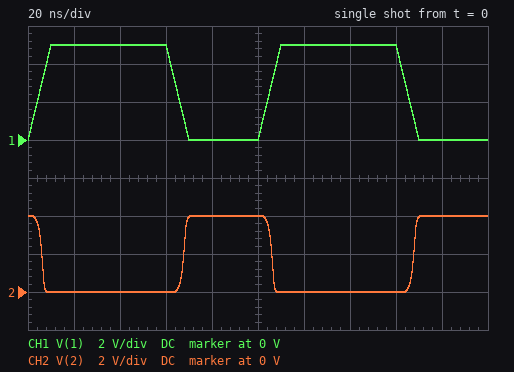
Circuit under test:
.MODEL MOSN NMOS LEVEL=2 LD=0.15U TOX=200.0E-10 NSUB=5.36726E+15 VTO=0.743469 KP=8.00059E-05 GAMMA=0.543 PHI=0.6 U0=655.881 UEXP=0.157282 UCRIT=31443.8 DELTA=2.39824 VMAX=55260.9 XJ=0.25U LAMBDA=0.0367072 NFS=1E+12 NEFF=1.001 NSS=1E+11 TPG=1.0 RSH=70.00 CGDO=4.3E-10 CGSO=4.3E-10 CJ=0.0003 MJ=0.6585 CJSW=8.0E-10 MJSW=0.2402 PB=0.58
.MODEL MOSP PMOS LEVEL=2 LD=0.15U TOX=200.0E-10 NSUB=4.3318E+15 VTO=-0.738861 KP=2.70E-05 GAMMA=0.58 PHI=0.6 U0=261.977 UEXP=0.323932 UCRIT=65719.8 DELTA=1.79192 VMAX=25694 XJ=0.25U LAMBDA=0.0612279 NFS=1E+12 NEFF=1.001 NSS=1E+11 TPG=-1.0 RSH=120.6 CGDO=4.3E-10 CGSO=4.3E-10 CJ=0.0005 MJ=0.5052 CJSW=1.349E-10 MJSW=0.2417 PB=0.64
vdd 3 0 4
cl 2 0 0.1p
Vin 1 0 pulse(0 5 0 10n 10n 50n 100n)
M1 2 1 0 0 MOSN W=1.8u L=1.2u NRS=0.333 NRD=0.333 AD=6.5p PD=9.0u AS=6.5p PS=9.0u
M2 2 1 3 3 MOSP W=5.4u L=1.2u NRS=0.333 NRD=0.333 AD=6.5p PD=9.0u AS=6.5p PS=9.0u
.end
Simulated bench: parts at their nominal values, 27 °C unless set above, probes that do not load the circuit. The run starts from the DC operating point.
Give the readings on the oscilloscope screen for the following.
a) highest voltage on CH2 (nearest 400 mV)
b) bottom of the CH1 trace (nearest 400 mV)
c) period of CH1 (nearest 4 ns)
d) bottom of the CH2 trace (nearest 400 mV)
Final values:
4.0 V
0 V
100 ns
0 V
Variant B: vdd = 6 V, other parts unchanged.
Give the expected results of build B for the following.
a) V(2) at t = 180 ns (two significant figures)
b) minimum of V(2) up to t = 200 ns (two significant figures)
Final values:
6.0 V
54 mV
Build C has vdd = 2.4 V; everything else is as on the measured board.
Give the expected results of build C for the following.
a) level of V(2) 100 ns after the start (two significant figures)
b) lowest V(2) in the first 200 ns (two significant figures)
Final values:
2.4 V
-13 mV
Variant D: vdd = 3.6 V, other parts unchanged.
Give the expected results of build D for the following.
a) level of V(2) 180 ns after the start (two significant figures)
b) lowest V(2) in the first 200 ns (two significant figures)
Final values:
3.6 V
-8.2 mV
